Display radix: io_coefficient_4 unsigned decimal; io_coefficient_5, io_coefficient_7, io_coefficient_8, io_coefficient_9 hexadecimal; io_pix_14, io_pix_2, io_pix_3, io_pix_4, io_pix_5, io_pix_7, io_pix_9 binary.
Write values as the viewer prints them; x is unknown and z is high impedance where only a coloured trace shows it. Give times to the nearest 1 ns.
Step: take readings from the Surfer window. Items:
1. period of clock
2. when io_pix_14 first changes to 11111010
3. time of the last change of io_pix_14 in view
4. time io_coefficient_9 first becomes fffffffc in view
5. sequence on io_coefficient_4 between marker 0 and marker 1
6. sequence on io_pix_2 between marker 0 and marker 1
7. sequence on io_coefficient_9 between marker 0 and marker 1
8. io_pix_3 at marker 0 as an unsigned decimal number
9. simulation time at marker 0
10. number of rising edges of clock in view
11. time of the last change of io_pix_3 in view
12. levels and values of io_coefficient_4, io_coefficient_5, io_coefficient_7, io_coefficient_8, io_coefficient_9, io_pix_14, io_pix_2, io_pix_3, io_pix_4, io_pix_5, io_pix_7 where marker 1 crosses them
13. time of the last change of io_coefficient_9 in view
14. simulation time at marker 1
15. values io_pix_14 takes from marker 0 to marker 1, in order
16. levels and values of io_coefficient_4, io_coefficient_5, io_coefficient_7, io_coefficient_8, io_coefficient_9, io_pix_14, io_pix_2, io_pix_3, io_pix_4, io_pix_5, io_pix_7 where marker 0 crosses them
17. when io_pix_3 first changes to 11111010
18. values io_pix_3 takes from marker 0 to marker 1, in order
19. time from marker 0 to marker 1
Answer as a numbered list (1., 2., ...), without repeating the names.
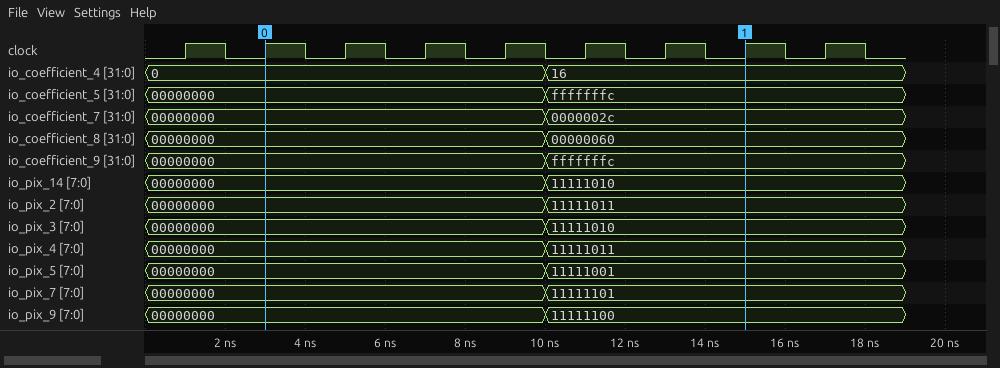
1. 2 ns
2. 10 ns
3. 10 ns
4. 10 ns
5. 0, 16
6. 00000000, 11111011
7. 00000000, fffffffc
8. 0
9. 3 ns
10. 9
11. 10 ns
12. io_coefficient_4=16, io_coefficient_5=fffffffc, io_coefficient_7=0000002c, io_coefficient_8=00000060, io_coefficient_9=fffffffc, io_pix_14=11111010, io_pix_2=11111011, io_pix_3=11111010, io_pix_4=11111011, io_pix_5=11111001, io_pix_7=11111101
13. 10 ns
14. 15 ns
15. 00000000, 11111010
16. io_coefficient_4=0, io_coefficient_5=00000000, io_coefficient_7=00000000, io_coefficient_8=00000000, io_coefficient_9=00000000, io_pix_14=00000000, io_pix_2=00000000, io_pix_3=00000000, io_pix_4=00000000, io_pix_5=00000000, io_pix_7=00000000
17. 10 ns
18. 00000000, 11111010
19. 12 ns
